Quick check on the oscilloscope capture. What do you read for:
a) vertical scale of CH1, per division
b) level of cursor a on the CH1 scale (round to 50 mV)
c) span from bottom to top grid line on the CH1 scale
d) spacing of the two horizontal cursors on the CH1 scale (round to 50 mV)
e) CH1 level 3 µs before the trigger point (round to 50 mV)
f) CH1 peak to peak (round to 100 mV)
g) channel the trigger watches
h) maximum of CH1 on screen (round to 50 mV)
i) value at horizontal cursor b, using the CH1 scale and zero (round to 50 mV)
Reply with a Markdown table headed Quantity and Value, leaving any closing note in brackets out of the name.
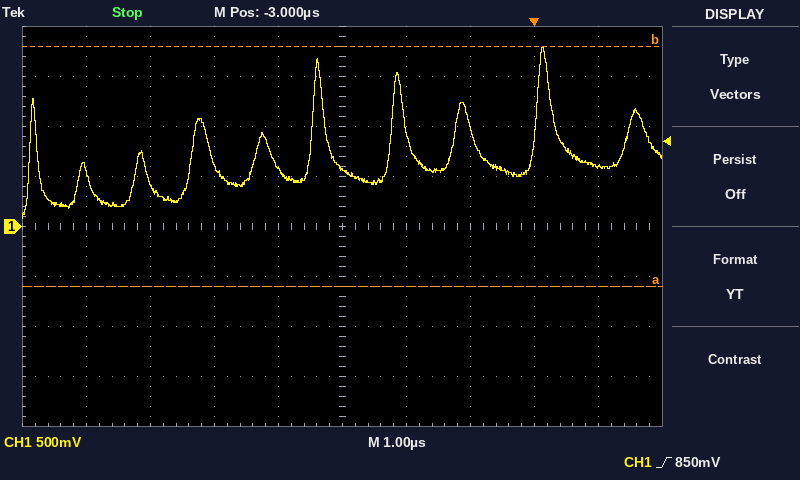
| Quantity | Value |
|---|---|
| vertical scale of CH1, per division | 500 mV |
| level of cursor a on the CH1 scale | -600 mV |
| span from bottom to top grid line on the CH1 scale | 4 V |
| spacing of the two horizontal cursors on the CH1 scale | 2.40 V |
| CH1 level 3 µs before the trigger point | 600 mV |
| CH1 peak to peak | 1.70 V |
| channel the trigger watches | CH1 |
| maximum of CH1 on screen | 1.80 V |
| value at horizontal cursor b, using the CH1 scale and zero | 1.80 V |
